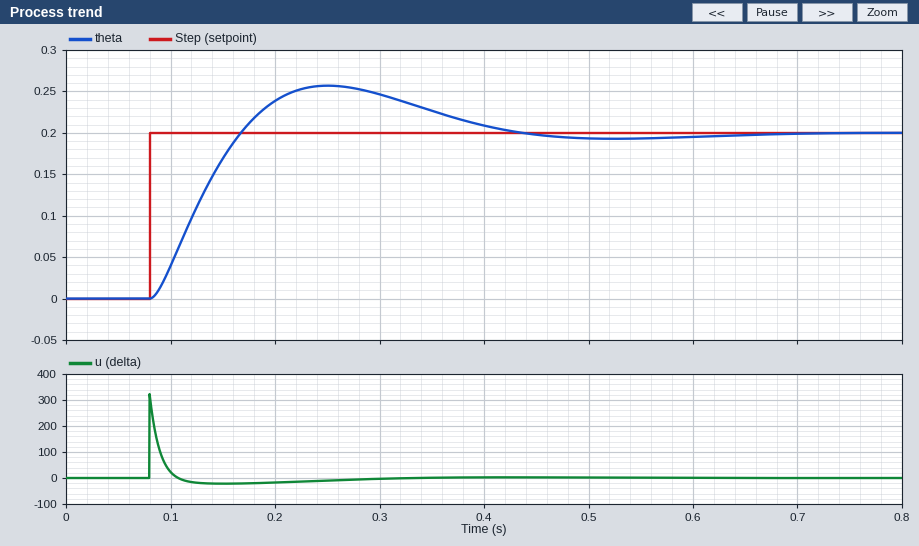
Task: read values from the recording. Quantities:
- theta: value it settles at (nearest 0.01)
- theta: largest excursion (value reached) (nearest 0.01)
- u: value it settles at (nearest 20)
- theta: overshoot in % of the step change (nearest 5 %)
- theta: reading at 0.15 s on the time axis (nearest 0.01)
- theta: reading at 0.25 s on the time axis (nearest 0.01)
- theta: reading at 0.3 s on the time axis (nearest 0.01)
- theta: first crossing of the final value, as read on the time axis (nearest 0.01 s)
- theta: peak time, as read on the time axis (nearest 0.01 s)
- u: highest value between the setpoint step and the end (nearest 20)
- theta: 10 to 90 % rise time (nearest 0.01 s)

0.20
0.26
0
30 %
0.17
0.26
0.25
0.17 s
0.25 s
320
0.06 s
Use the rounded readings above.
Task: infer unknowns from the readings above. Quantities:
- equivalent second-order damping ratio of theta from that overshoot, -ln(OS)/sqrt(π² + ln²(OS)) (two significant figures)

0.36
